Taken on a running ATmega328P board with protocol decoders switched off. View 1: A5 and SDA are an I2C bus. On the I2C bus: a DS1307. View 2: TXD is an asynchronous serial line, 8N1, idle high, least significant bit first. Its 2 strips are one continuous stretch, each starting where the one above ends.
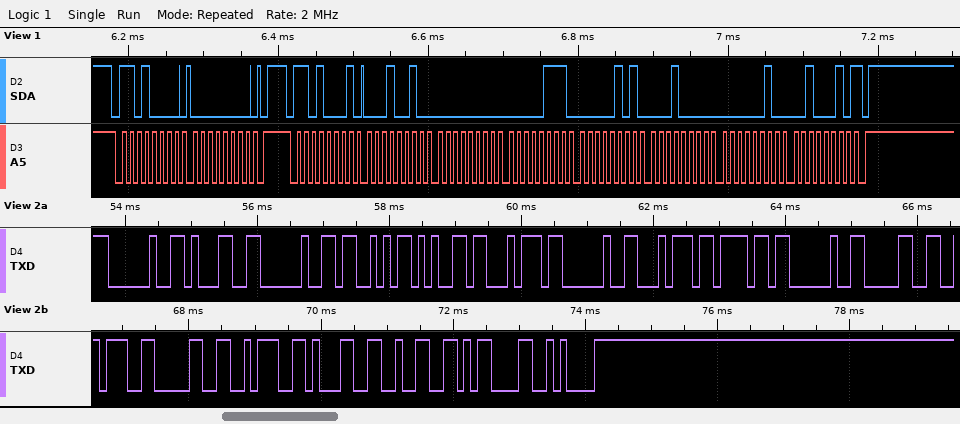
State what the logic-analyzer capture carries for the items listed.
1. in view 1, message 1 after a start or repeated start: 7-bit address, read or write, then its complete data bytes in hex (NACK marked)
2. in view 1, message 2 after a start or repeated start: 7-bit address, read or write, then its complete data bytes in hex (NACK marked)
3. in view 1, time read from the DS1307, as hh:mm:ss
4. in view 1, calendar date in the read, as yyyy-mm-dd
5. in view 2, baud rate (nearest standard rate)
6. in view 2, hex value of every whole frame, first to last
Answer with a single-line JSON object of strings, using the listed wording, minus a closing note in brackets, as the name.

{"in view 1, message 1 after a start or repeated start: 7-bit address, read or write, then its complete data bytes in hex": "0x68 write: 00", "in view 1, message 2 after a start or repeated start: 7-bit address, read or write, then its complete data bytes in hex": "0x68 read: 12 00 07 05 10 02 22 NACK", "in view 1, time read from the DS1307, as hh:mm:ss": "07:00:12", "in view 1, calendar date in the read, as yyyy-mm-dd": "2022-02-10", "in view 2, baud rate": "9600 baud", "in view 2, hex value of every whole frame, first to last": "20 31 20 53 65 74 20 74 6F 20 30 3A 30 3A 31 32 0D 0A"}
